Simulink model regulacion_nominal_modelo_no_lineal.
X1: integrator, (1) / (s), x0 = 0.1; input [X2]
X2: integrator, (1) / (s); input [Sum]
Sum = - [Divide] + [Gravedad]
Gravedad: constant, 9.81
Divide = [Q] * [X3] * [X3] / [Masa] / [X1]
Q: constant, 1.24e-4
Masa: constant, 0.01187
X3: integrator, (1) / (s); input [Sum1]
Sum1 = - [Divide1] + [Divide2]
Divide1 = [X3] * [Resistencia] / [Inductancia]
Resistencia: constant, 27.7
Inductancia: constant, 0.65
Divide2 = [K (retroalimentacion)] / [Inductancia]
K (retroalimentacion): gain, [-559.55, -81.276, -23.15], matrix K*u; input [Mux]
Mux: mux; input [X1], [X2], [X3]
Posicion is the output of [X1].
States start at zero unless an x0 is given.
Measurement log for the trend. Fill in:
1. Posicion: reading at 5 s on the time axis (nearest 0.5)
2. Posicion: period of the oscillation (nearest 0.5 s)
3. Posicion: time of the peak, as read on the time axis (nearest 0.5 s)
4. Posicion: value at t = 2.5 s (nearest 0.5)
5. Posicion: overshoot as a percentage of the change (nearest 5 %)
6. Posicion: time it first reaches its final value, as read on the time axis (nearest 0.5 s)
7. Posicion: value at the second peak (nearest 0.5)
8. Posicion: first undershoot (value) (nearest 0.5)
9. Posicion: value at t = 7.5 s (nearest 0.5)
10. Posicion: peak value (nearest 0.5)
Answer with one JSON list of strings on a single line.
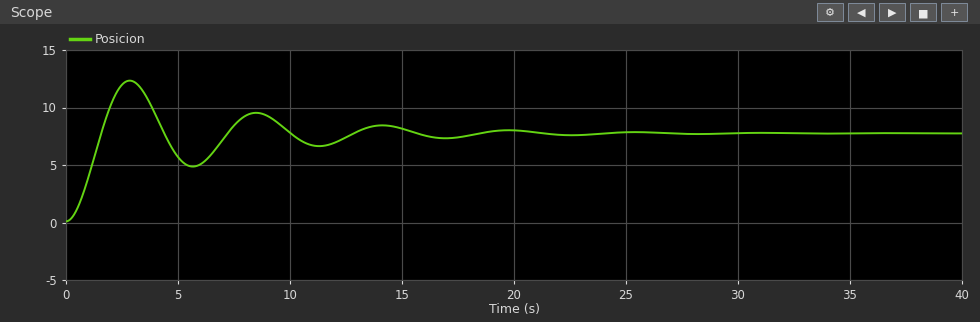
["5.5", "5.5 s", "3.0 s", "12.0", "60 %", "1.5 s", "9.5", "5.0", "8.5", "12.5"]
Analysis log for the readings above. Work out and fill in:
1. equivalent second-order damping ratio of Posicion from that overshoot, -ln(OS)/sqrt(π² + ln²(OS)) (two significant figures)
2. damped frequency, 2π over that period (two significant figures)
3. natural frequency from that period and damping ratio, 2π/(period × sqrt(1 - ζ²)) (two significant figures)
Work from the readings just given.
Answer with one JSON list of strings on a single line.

["0.16", "1.1 rad/s", "1.2 rad/s"]
